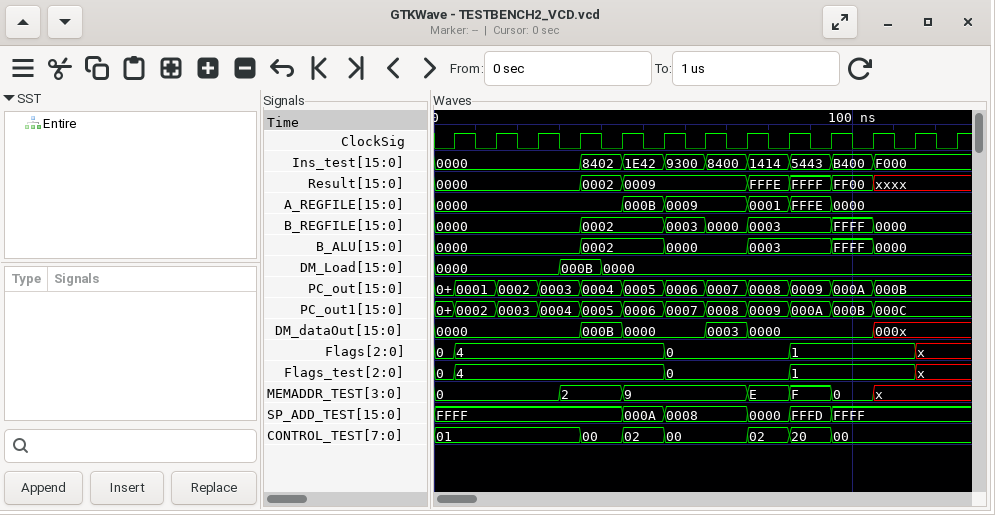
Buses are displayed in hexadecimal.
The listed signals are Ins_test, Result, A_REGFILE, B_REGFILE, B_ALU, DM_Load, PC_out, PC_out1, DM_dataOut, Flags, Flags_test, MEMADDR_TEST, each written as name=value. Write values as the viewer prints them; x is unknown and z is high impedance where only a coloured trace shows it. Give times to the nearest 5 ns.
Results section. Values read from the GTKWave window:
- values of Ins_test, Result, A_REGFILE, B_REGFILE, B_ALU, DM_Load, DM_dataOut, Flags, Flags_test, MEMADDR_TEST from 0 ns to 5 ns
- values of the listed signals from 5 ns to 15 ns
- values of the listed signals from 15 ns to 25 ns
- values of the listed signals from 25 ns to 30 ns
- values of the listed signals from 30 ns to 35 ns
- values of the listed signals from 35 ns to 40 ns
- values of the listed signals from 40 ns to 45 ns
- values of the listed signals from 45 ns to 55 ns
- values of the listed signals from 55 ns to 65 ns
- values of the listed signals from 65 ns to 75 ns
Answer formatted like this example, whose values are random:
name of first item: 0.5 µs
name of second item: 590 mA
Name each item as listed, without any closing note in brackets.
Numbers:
values of Ins_test, Result, A_REGFILE, B_REGFILE, B_ALU, DM_Load, DM_dataOut, Flags, Flags_test, MEMADDR_TEST from 0 ns to 5 ns: Ins_test=0000, Result=0000, A_REGFILE=0000, B_REGFILE=0000, B_ALU=0000, DM_Load=0000, DM_dataOut=0000, Flags=0, Flags_test=0, MEMADDR_TEST=0
values of the listed signals from 5 ns to 15 ns: Ins_test=0000, Result=0000, A_REGFILE=0000, B_REGFILE=0000, B_ALU=0000, DM_Load=0000, PC_out=0001, PC_out1=0002, DM_dataOut=0000, Flags=4, Flags_test=4, MEMADDR_TEST=0
values of the listed signals from 15 ns to 25 ns: Ins_test=0000, Result=0000, A_REGFILE=0000, B_REGFILE=0000, B_ALU=0000, DM_Load=0000, PC_out=0002, PC_out1=0003, DM_dataOut=0000, Flags=4, Flags_test=4, MEMADDR_TEST=0
values of the listed signals from 25 ns to 30 ns: Ins_test=0000, Result=0000, A_REGFILE=0000, B_REGFILE=0000, B_ALU=0000, DM_Load=0000, PC_out=0003, PC_out1=0004, DM_dataOut=0000, Flags=4, Flags_test=4, MEMADDR_TEST=0
values of the listed signals from 30 ns to 35 ns: Ins_test=0000, Result=0000, A_REGFILE=0000, B_REGFILE=0000, B_ALU=0000, DM_Load=000B, PC_out=0003, PC_out1=0004, DM_dataOut=0000, Flags=4, Flags_test=4, MEMADDR_TEST=2
values of the listed signals from 35 ns to 40 ns: Ins_test=8402, Result=0002, A_REGFILE=0000, B_REGFILE=0002, B_ALU=0002, DM_Load=000B, PC_out=0004, PC_out1=0005, DM_dataOut=000B, Flags=4, Flags_test=4, MEMADDR_TEST=2
values of the listed signals from 40 ns to 45 ns: Ins_test=8402, Result=0002, A_REGFILE=0000, B_REGFILE=0002, B_ALU=0002, DM_Load=0000, PC_out=0004, PC_out1=0005, DM_dataOut=000B, Flags=4, Flags_test=4, MEMADDR_TEST=2
values of the listed signals from 45 ns to 55 ns: Ins_test=1E42, Result=0009, A_REGFILE=000B, B_REGFILE=0002, B_ALU=0002, DM_Load=0000, PC_out=0005, PC_out1=0006, DM_dataOut=0000, Flags=4, Flags_test=4, MEMADDR_TEST=9
values of the listed signals from 55 ns to 65 ns: Ins_test=9300, Result=0009, A_REGFILE=0009, B_REGFILE=0003, B_ALU=0000, DM_Load=0000, PC_out=0006, PC_out1=0007, DM_dataOut=0000, Flags=0, Flags_test=0, MEMADDR_TEST=9
values of the listed signals from 65 ns to 75 ns: Ins_test=8400, Result=0009, A_REGFILE=0009, B_REGFILE=0000, B_ALU=0000, DM_Load=0000, PC_out=0007, PC_out1=0008, DM_dataOut=0003, Flags=0, Flags_test=0, MEMADDR_TEST=9
